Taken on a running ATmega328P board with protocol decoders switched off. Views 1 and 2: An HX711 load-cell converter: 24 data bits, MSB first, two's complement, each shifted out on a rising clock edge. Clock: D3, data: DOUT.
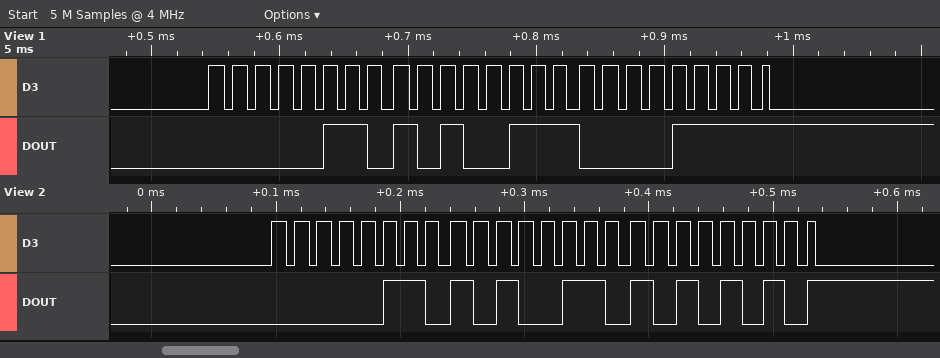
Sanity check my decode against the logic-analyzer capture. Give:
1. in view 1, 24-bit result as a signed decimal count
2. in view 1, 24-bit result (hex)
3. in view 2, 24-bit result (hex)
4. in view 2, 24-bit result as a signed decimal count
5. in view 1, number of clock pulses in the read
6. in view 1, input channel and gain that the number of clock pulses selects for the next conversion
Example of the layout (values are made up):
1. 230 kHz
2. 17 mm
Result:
1. 435983
2. 0x06A70F
3. 0x06A6AA
4. 435882
5. 25
6. channel A, gain 128
